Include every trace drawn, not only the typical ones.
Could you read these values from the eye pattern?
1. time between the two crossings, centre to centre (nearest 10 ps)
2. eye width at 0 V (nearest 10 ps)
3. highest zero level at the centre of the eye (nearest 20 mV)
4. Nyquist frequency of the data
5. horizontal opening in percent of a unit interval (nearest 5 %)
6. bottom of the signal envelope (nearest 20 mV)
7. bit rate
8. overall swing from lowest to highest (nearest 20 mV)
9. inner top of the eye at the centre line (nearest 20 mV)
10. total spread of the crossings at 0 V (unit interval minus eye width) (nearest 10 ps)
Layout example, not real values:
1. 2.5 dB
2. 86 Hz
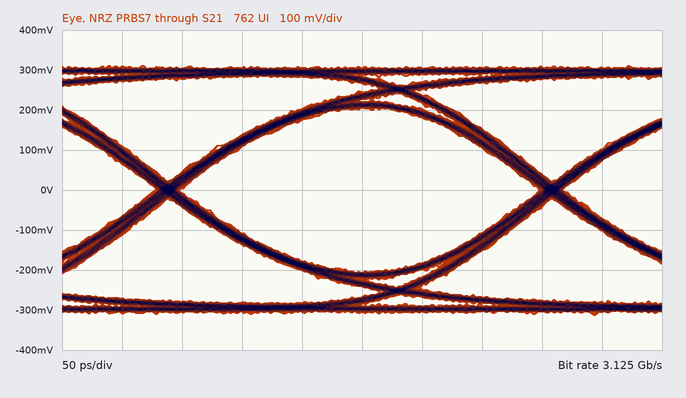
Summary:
1. 320 ps
2. 300 ps
3. -200 mV
4. 1.5625 GHz
5. 95 %
6. -320 mV
7. 3.125 Gb/s
8. 620 mV
9. 200 mV
10. 20 ps
